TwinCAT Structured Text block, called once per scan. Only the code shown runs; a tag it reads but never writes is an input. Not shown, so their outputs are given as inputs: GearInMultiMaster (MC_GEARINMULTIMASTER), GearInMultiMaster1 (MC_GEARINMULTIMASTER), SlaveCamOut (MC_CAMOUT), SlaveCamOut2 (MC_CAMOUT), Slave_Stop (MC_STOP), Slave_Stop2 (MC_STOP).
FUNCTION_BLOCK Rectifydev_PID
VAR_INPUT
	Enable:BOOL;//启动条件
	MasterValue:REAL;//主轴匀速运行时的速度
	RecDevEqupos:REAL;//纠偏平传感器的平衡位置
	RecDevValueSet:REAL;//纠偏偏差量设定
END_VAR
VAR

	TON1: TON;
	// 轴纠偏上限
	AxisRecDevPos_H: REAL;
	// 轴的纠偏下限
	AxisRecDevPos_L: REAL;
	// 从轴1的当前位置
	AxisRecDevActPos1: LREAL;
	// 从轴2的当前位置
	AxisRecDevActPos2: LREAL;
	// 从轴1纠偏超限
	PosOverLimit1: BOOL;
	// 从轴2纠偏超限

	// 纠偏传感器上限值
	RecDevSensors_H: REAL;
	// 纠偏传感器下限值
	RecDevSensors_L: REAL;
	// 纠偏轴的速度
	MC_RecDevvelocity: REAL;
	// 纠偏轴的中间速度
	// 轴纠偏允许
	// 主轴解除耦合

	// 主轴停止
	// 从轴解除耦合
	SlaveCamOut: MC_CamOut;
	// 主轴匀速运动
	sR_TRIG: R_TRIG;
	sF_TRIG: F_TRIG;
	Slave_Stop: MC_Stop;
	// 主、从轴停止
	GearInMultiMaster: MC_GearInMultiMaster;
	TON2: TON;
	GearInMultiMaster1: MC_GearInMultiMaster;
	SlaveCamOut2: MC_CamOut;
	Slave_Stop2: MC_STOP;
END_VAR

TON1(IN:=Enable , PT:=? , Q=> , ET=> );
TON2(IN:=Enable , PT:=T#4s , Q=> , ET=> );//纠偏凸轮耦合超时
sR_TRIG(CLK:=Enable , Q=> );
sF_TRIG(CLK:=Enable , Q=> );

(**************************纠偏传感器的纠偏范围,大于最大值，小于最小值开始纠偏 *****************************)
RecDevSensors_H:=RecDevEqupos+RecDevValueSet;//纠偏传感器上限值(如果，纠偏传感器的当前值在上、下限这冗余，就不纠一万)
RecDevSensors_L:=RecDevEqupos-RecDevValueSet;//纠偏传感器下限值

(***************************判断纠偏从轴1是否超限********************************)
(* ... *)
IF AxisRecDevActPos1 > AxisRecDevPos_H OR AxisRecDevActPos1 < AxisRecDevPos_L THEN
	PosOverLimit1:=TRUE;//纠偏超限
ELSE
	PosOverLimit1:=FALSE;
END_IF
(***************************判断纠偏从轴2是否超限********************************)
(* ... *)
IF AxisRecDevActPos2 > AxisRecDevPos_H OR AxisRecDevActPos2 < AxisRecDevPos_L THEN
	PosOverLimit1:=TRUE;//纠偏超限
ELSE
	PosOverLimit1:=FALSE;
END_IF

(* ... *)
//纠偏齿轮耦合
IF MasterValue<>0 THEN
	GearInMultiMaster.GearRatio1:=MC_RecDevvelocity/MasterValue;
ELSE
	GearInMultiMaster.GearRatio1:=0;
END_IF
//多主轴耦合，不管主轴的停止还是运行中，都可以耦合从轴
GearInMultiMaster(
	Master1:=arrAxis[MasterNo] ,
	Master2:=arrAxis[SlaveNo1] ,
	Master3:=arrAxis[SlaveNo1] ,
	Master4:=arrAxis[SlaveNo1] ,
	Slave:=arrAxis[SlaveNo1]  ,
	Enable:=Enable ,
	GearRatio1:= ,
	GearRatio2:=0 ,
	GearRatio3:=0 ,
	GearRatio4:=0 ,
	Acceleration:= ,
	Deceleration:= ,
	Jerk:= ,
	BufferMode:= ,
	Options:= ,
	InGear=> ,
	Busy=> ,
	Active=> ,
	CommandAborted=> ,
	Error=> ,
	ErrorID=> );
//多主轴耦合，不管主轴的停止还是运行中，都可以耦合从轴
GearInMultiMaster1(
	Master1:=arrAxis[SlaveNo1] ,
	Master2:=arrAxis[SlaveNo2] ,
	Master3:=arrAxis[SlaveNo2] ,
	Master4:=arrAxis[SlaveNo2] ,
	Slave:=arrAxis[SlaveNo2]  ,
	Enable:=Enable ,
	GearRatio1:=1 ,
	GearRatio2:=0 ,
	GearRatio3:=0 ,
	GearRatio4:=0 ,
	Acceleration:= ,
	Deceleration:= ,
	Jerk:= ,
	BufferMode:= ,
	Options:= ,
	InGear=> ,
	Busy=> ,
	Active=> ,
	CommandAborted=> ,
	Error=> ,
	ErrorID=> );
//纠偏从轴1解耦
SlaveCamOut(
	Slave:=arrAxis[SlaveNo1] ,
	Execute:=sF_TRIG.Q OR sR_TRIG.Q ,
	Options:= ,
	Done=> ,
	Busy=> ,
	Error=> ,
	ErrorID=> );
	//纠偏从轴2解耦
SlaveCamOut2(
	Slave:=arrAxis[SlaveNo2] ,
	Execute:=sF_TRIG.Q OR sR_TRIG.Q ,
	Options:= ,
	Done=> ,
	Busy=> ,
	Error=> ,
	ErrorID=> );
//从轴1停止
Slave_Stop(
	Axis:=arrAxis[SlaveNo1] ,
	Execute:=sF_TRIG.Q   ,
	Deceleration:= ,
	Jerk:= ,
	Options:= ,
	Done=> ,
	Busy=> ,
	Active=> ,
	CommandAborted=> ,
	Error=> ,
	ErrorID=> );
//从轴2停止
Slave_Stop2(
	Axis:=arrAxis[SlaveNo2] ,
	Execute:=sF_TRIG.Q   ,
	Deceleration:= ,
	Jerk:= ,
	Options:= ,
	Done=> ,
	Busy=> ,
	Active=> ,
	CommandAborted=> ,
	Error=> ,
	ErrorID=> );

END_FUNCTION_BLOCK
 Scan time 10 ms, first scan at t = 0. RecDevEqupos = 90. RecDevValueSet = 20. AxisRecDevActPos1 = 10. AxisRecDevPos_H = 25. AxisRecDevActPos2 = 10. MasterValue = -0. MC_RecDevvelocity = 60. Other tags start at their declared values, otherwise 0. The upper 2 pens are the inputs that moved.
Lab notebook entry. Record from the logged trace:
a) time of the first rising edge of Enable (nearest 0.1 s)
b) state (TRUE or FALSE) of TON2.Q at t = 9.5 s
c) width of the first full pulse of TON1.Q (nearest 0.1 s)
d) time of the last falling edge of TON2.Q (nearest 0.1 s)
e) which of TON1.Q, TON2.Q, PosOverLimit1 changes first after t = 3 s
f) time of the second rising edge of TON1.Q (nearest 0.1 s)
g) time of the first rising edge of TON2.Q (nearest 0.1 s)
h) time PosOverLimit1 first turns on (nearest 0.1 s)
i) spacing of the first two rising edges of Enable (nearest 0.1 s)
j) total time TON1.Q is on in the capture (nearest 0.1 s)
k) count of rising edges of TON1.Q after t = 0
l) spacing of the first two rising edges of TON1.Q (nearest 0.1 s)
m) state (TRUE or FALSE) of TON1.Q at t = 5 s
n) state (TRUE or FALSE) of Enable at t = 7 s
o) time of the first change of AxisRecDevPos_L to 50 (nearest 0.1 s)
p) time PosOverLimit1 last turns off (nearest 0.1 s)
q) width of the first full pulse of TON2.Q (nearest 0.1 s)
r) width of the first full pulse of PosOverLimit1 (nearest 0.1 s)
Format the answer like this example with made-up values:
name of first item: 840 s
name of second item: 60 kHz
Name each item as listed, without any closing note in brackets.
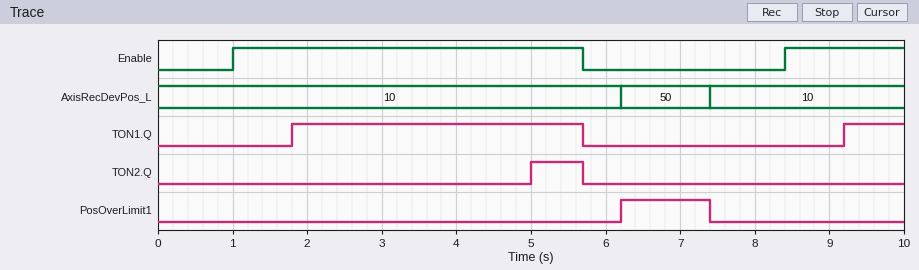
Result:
time of the first rising edge of Enable: 1.0 s
state (TRUE or FALSE) of TON2.Q at t = 9.5 s: FALSE
width of the first full pulse of TON1.Q: 3.9 s
time of the last falling edge of TON2.Q: 5.7 s
which of TON1.Q, TON2.Q, PosOverLimit1 changes first after t = 3 s: TON2.Q
time of the second rising edge of TON1.Q: 9.2 s
time of the first rising edge of TON2.Q: 5.0 s
time PosOverLimit1 first turns on: 6.2 s
spacing of the first two rising edges of Enable: 7.4 s
total time TON1.Q is on in the capture: 4.7 s
count of rising edges of TON1.Q after t = 0: 2
spacing of the first two rising edges of TON1.Q: 7.4 s
state (TRUE or FALSE) of TON1.Q at t = 5 s: TRUE
state (TRUE or FALSE) of Enable at t = 7 s: FALSE
time of the first change of AxisRecDevPos_L to 50: 6.2 s
time PosOverLimit1 last turns off: 7.4 s
width of the first full pulse of TON2.Q: 0.7 s
width of the first full pulse of PosOverLimit1: 1.2 s
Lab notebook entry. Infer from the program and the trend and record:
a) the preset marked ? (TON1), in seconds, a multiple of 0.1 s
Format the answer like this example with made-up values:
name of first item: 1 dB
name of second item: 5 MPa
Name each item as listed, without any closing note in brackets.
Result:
the preset marked ? (TON1), in seconds, a multiple of 0.1 s: 0.8 s
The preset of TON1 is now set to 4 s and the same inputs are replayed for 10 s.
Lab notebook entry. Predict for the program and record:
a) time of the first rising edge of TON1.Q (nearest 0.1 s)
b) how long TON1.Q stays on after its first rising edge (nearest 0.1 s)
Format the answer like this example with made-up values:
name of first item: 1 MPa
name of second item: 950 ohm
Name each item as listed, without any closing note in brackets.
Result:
time of the first rising edge of TON1.Q: 5.0 s
how long TON1.Q stays on after its first rising edge: 0.7 s
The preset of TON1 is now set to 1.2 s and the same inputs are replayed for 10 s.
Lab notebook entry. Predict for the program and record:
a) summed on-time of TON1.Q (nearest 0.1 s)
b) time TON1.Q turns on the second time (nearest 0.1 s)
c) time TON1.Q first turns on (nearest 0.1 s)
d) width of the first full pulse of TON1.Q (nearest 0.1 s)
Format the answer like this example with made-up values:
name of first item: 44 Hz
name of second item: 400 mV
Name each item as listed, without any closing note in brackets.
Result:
summed on-time of TON1.Q: 3.9 s
time TON1.Q turns on the second time: 9.6 s
time TON1.Q first turns on: 2.2 s
width of the first full pulse of TON1.Q: 3.5 s
